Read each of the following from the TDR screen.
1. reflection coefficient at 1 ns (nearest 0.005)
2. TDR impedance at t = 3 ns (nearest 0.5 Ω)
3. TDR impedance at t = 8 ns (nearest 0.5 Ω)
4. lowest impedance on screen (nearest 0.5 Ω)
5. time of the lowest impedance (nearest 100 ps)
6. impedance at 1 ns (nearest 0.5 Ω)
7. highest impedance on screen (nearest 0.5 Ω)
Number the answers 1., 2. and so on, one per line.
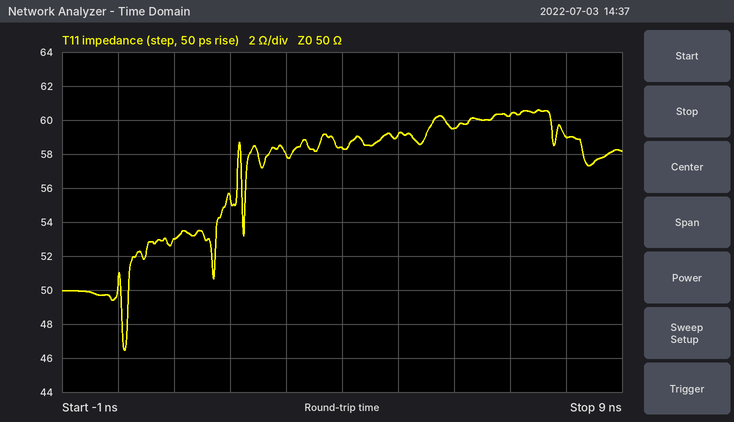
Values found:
1. +0.030
2. 58.0 Ω
3. 59.0 Ω
4. 46.5 Ω
5. 100 ps
6. 53.0 Ω
7. 60.5 Ω
